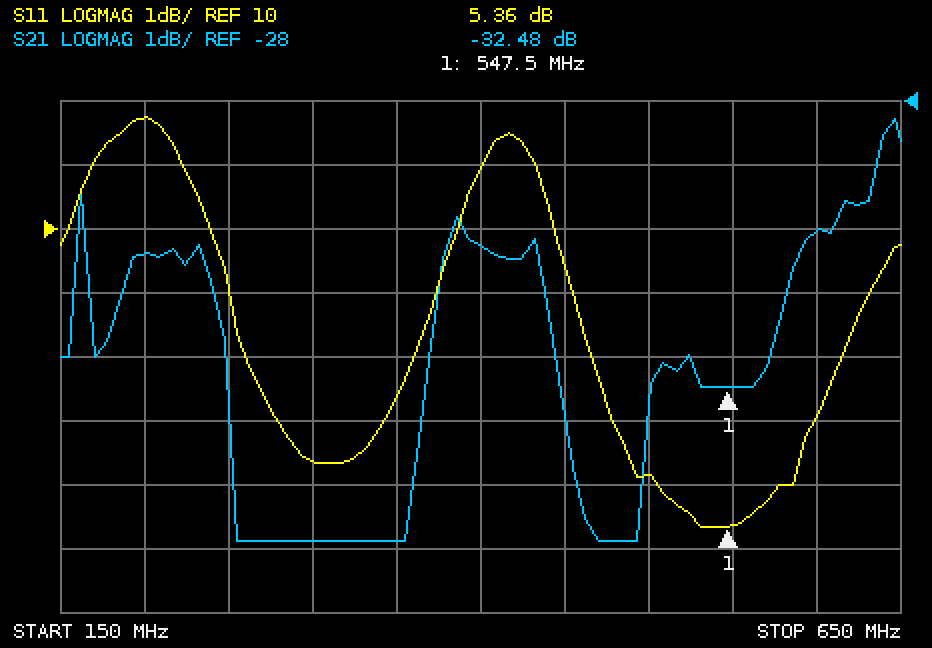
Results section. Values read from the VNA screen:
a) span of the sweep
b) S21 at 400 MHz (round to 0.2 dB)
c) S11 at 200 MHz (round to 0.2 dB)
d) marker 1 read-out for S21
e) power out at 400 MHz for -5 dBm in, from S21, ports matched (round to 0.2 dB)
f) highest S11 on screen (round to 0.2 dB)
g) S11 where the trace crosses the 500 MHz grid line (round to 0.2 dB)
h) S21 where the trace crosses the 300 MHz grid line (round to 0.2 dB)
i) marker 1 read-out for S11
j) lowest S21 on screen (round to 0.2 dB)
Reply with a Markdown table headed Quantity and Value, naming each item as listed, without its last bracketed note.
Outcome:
| Quantity | Value |
|---|---|
| span of the sweep | 500 MHz |
| S21 at 400 MHz | -30.2 dB |
| S11 at 200 MHz | 11.8 dB |
| marker 1 read-out for S21 | -32.48 dB |
| power out at 400 MHz for -5 dBm in, from S21, ports matched | -35.2 dBm |
| highest S11 on screen | 11.8 dB |
| S11 where the trace crosses the 500 MHz grid line | 6.2 dB |
| S21 where the trace crosses the 300 MHz grid line | -34.8 dB |
| marker 1 read-out for S11 | 5.36 dB |
| lowest S21 on screen | -34.8 dB |
